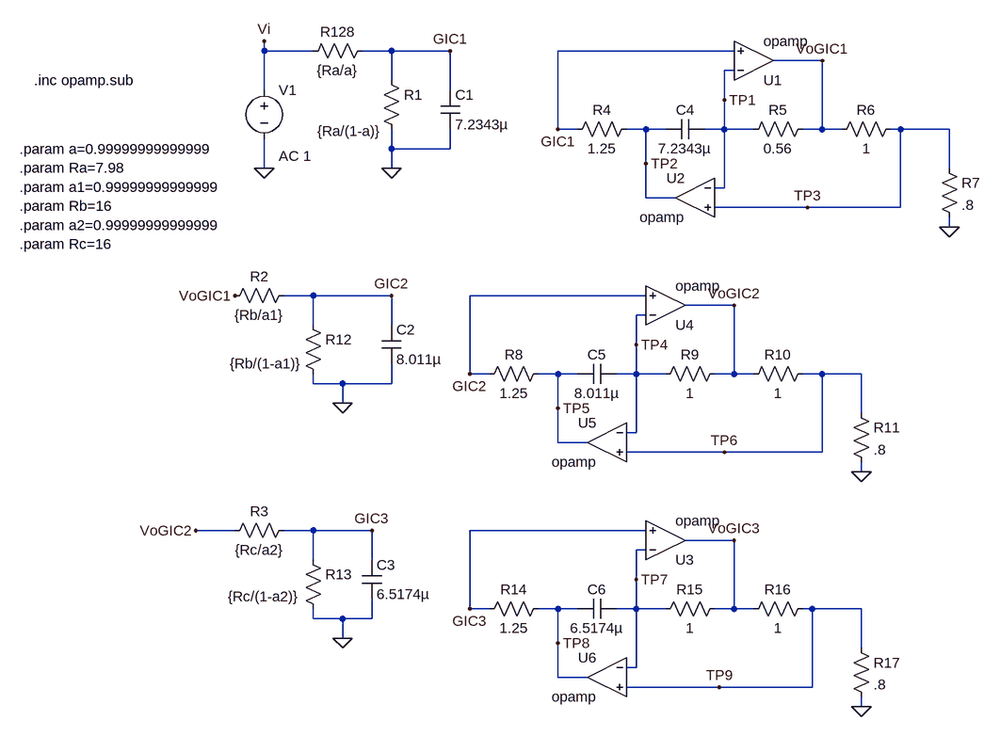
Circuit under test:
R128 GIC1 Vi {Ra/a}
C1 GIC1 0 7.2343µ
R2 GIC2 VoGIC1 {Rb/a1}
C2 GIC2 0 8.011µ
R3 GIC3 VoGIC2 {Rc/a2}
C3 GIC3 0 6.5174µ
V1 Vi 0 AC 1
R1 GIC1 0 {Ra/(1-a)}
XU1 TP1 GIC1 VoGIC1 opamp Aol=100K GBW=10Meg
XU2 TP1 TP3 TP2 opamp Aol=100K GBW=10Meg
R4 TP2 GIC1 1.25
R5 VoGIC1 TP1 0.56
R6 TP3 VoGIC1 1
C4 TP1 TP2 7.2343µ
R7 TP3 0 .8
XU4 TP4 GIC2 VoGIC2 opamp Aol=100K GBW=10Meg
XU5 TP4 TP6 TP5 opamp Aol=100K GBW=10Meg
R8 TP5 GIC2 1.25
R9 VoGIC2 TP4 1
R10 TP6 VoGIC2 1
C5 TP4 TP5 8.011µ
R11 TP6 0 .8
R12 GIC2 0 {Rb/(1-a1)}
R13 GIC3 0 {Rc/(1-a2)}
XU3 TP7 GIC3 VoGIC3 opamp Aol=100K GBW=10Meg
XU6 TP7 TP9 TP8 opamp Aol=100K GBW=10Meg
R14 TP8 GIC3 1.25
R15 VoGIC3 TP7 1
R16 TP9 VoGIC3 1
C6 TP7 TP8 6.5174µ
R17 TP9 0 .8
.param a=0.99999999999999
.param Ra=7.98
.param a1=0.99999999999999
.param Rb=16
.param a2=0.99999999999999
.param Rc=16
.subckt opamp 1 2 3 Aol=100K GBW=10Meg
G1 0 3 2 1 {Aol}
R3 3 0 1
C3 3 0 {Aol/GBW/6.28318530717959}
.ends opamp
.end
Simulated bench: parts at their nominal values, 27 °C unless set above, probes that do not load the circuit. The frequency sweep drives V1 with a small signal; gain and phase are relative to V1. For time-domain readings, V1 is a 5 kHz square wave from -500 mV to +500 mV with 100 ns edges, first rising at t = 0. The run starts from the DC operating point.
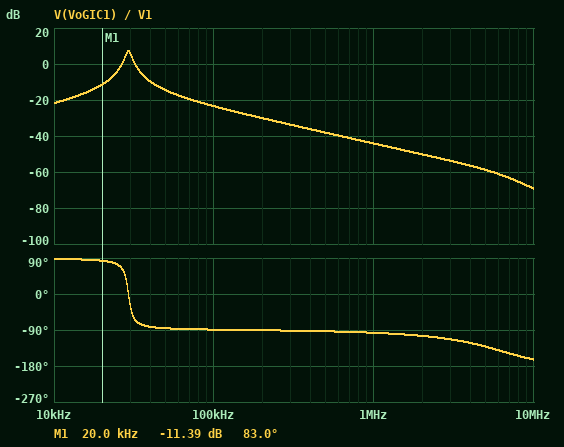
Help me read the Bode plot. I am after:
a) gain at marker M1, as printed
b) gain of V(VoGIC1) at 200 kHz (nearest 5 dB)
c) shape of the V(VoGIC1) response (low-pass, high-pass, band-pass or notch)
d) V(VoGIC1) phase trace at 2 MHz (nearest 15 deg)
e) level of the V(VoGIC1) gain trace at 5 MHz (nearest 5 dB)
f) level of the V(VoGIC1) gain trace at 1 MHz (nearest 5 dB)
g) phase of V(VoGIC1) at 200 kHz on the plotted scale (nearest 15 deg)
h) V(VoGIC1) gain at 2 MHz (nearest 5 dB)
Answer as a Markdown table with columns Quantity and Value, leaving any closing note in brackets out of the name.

| Quantity | Value |
|---|---|
| gain at marker M1, as printed | -11.39 dB |
| gain of V(VoGIC1) at 200 kHz | -30 dB |
| shape of the V(VoGIC1) response | band-pass |
| V(VoGIC1) phase trace at 2 MHz | -105 deg |
| level of the V(VoGIC1) gain trace at 5 MHz | -60 dB |
| level of the V(VoGIC1) gain trace at 1 MHz | -45 dB |
| phase of V(VoGIC1) at 200 kHz on the plotted scale | -90 deg |
| V(VoGIC1) gain at 2 MHz | -50 dB |
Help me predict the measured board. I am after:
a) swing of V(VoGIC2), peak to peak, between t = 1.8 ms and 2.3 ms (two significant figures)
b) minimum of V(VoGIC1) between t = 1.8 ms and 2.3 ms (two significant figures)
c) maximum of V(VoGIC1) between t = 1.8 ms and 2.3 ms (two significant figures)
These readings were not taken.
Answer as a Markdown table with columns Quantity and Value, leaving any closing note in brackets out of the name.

| Quantity | Value |
|---|---|
| swing of V(VoGIC2), peak to peak, between t = 1.8 ms and 2.3 ms | 71 mV |
| minimum of V(VoGIC1) between t = 1.8 ms and 2.3 ms | -140 mV |
| maximum of V(VoGIC1) between t = 1.8 ms and 2.3 ms | 140 mV |
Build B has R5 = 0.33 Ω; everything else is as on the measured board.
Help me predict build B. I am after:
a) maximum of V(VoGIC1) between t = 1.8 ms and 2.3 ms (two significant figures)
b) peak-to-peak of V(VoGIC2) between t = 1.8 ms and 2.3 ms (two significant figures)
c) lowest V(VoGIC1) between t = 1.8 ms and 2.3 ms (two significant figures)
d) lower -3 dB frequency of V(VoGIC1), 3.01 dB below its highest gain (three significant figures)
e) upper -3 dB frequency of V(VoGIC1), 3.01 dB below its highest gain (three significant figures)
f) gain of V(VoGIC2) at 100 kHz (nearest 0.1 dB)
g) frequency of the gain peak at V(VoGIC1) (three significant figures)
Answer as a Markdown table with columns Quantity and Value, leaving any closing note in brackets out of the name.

| Quantity | Value |
|---|---|
| maximum of V(VoGIC1) between t = 1.8 ms and 2.3 ms | 130 mV |
| peak-to-peak of V(VoGIC2) between t = 1.8 ms and 2.3 ms | 40 mV |
| lowest V(VoGIC1) between t = 1.8 ms and 2.3 ms | -130 mV |
| lower -3 dB frequency of V(VoGIC1), 3.01 dB below its highest gain | 36.6 kHz |
| upper -3 dB frequency of V(VoGIC1), 3.01 dB below its highest gain | 39.3 kHz |
| gain of V(VoGIC2) at 100 kHz | -53.7 dB |
| frequency of the gain peak at V(VoGIC1) | 37.9 kHz |
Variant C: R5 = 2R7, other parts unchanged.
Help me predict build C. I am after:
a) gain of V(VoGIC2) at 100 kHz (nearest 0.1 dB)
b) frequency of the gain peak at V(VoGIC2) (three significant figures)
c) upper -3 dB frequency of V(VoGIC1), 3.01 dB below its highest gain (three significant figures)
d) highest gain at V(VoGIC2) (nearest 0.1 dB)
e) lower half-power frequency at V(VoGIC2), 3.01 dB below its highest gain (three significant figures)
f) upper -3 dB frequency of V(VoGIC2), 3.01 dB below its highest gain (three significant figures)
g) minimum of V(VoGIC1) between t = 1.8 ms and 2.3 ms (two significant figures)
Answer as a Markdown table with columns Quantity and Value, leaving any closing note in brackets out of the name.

| Quantity | Value |
|---|---|
| gain of V(VoGIC2) at 100 kHz | -54.8 dB |
| frequency of the gain peak at V(VoGIC2) | 19.7 kHz |
| upper -3 dB frequency of V(VoGIC1), 3.01 dB below its highest gain | 14.8 kHz |
| highest gain at V(VoGIC2) | 2.0 dB |
| lower half-power frequency at V(VoGIC2), 3.01 dB below its highest gain | 19.1 kHz |
| upper -3 dB frequency of V(VoGIC2), 3.01 dB below its highest gain | 20.3 kHz |
| minimum of V(VoGIC1) between t = 1.8 ms and 2.3 ms | -430 mV |
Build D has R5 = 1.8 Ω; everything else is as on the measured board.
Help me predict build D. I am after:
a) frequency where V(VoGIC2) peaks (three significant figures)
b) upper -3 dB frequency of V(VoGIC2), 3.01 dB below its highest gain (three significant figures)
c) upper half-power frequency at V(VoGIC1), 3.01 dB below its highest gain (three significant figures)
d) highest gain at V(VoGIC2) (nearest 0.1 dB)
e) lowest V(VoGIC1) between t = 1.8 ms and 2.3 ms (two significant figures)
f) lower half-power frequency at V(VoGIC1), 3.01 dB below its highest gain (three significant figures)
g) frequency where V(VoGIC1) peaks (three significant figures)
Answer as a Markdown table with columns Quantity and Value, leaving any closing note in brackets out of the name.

| Quantity | Value |
|---|---|
| frequency where V(VoGIC2) peaks | 19.7 kHz |
| upper -3 dB frequency of V(VoGIC2), 3.01 dB below its highest gain | 20.3 kHz |
| upper half-power frequency at V(VoGIC1), 3.01 dB below its highest gain | 17.8 kHz |
| highest gain at V(VoGIC2) | 6.3 dB |
| lowest V(VoGIC1) between t = 1.8 ms and 2.3 ms | -450 mV |
| lower half-power frequency at V(VoGIC1), 3.01 dB below its highest gain | 15.0 kHz |
| frequency where V(VoGIC1) peaks | 16.3 kHz |
